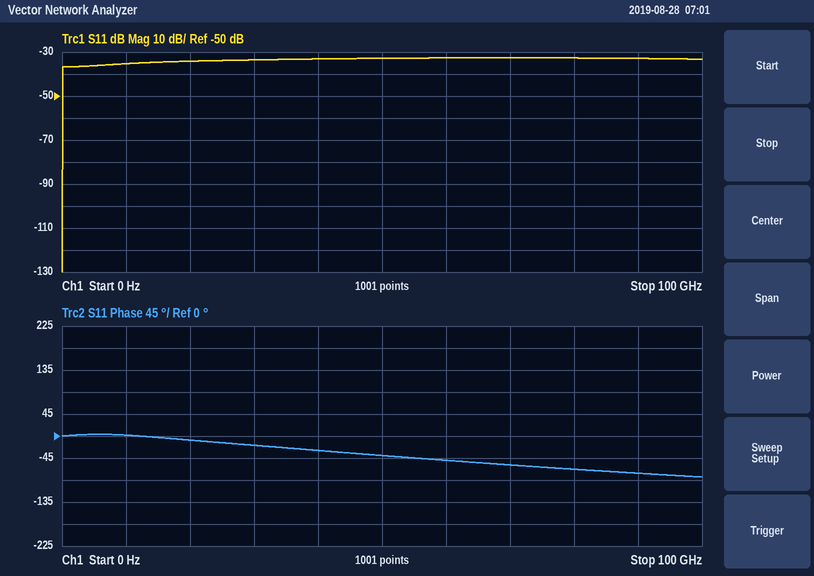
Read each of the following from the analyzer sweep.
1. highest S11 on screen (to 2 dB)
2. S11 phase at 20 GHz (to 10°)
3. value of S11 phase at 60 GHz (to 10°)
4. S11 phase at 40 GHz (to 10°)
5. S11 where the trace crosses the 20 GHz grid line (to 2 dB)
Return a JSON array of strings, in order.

["-32 dB", "-10°", "-50°", "-30°", "-34 dB"]
